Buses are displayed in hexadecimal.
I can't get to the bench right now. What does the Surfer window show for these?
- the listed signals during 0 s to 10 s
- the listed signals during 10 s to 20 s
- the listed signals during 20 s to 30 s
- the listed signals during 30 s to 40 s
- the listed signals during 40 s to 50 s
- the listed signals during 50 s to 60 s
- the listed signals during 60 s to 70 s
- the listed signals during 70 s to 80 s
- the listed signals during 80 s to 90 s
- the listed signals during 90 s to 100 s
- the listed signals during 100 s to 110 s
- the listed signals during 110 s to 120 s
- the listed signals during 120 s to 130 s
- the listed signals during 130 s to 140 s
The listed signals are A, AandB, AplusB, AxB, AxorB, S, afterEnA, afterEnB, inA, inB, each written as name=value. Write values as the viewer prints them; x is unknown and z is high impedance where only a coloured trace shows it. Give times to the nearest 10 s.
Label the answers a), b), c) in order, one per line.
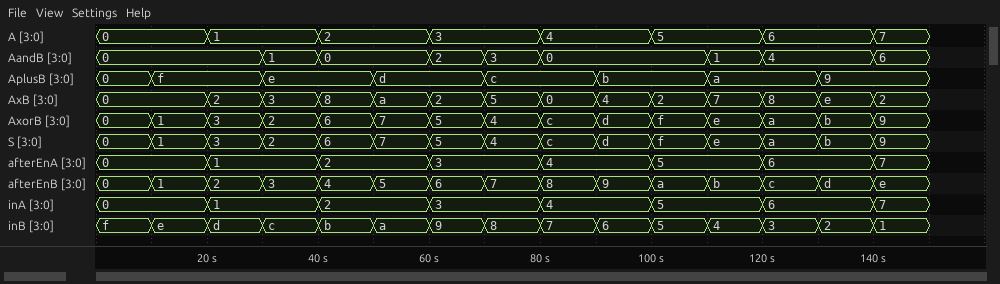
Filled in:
a) A=0, AandB=0, AplusB=0, AxB=0, AxorB=0, S=0, afterEnA=0, afterEnB=0, inA=0, inB=f
b) A=0, AandB=0, AplusB=f, AxB=0, AxorB=1, S=1, afterEnA=0, afterEnB=1, inA=0, inB=e
c) A=1, AandB=0, AplusB=f, AxB=2, AxorB=3, S=3, afterEnA=1, afterEnB=2, inA=1, inB=d
d) A=1, AandB=1, AplusB=e, AxB=3, AxorB=2, S=2, afterEnA=1, afterEnB=3, inA=1, inB=c
e) A=2, AandB=0, AplusB=e, AxB=8, AxorB=6, S=6, afterEnA=2, afterEnB=4, inA=2, inB=b
f) A=2, AandB=0, AplusB=d, AxB=a, AxorB=7, S=7, afterEnA=2, afterEnB=5, inA=2, inB=a
g) A=3, AandB=2, AplusB=d, AxB=2, AxorB=5, S=5, afterEnA=3, afterEnB=6, inA=3, inB=9
h) A=3, AandB=3, AplusB=c, AxB=5, AxorB=4, S=4, afterEnA=3, afterEnB=7, inA=3, inB=8
i) A=4, AandB=0, AplusB=c, AxB=0, AxorB=c, S=c, afterEnA=4, afterEnB=8, inA=4, inB=7
j) A=4, AandB=0, AplusB=b, AxB=4, AxorB=d, S=d, afterEnA=4, afterEnB=9, inA=4, inB=6
k) A=5, AandB=0, AplusB=b, AxB=2, AxorB=f, S=f, afterEnA=5, afterEnB=a, inA=5, inB=5
l) A=5, AandB=1, AplusB=a, AxB=7, AxorB=e, S=e, afterEnA=5, afterEnB=b, inA=5, inB=4
m) A=6, AandB=4, AplusB=a, AxB=8, AxorB=a, S=a, afterEnA=6, afterEnB=c, inA=6, inB=3
n) A=6, AandB=4, AplusB=9, AxB=e, AxorB=b, S=b, afterEnA=6, afterEnB=d, inA=6, inB=2
